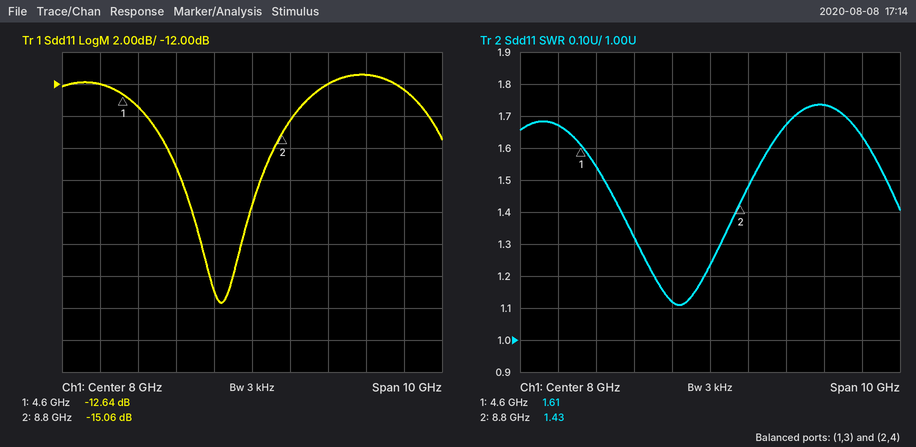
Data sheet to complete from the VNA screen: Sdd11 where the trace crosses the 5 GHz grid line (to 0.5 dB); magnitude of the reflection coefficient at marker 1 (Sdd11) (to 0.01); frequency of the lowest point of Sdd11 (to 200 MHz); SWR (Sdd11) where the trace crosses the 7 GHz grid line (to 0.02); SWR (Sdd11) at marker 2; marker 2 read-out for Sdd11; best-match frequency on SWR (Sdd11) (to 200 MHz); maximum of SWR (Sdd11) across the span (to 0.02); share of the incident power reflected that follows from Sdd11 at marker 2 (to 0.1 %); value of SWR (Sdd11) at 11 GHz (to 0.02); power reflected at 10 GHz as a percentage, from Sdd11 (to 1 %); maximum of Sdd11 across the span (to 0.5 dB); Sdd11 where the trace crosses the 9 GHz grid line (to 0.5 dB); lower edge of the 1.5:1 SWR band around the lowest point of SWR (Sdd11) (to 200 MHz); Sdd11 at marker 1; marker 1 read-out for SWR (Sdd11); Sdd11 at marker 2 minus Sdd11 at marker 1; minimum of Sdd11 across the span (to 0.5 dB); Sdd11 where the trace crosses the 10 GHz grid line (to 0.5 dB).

-13.5 dB
0.23
7.2 GHz
1.12
1.43
-15.06 dB
7.2 GHz
1.74
3.1 %
1.74
6 %
-11.5 dB
-14.5 dB
5.2 GHz
-12.64 dB
1.61
-2.42 dB
-25.5 dB
-12.0 dB
